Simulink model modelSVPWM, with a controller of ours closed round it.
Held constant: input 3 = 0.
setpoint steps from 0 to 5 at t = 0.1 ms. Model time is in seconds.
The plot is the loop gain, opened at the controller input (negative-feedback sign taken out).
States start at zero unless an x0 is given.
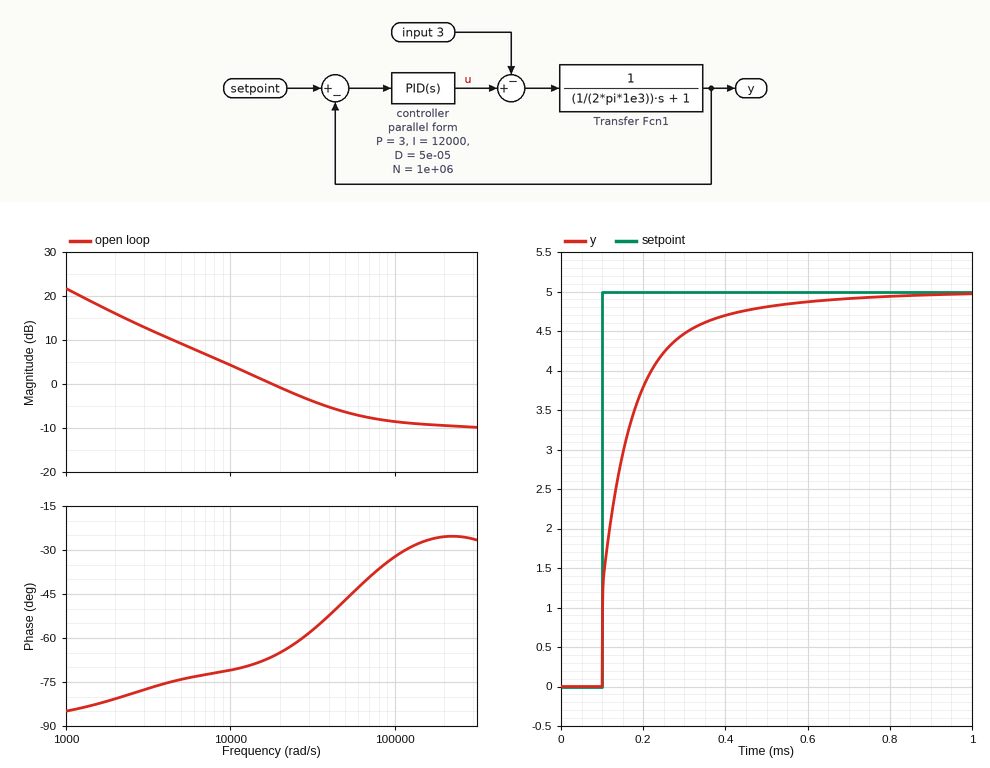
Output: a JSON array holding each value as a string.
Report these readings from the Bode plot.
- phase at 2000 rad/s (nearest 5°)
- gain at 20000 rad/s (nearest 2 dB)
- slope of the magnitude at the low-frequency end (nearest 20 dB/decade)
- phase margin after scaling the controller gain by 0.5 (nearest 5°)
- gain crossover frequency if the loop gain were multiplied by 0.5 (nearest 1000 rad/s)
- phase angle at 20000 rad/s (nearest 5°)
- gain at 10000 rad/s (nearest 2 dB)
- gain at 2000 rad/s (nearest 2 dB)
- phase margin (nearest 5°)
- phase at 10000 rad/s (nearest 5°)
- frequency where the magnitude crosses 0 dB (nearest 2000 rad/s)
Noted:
["-80°", "0 dB", "-20 dB/decade", "110°", "8000 rad/s", "-65°", "4 dB", "16 dB", "115°", "-70°", "18000 rad/s"]
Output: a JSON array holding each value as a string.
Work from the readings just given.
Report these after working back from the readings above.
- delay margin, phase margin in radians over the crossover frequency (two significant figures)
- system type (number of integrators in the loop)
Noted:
["0.00011 s", "1"]
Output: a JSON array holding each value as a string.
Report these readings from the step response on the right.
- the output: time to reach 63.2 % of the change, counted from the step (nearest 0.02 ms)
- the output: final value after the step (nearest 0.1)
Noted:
["0.06 ms", "5.0"]
